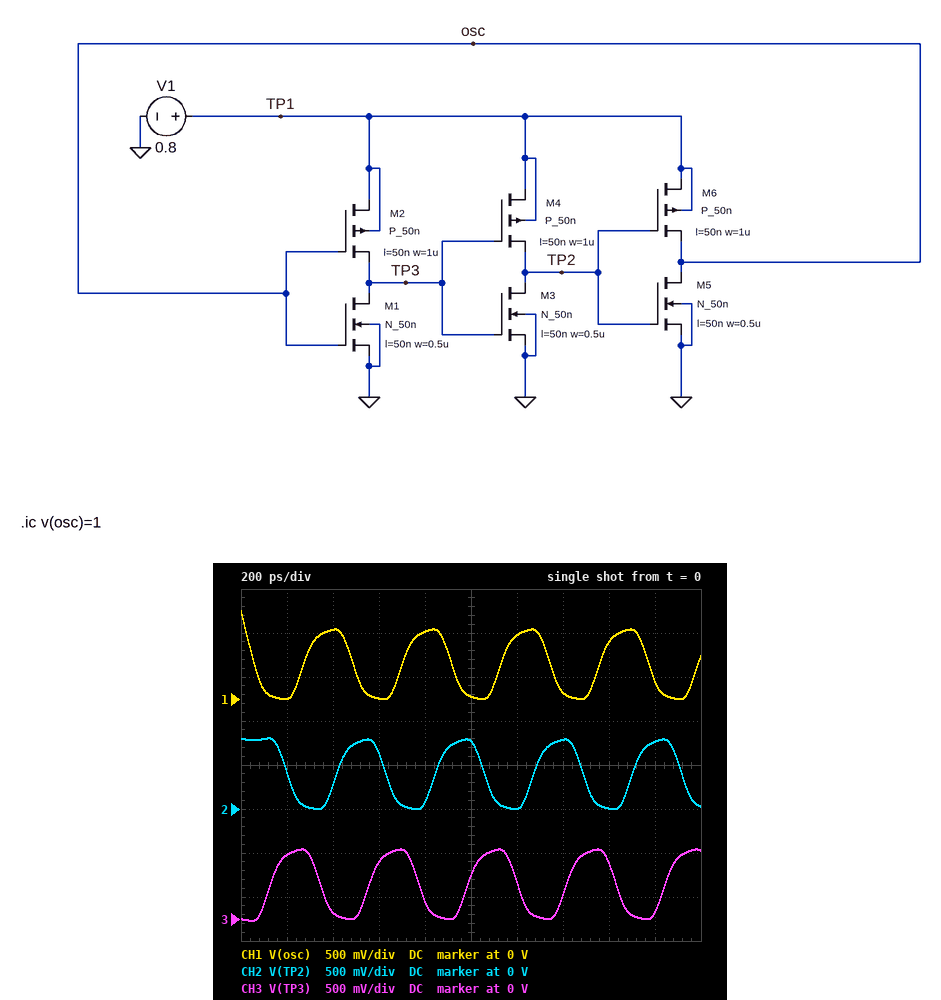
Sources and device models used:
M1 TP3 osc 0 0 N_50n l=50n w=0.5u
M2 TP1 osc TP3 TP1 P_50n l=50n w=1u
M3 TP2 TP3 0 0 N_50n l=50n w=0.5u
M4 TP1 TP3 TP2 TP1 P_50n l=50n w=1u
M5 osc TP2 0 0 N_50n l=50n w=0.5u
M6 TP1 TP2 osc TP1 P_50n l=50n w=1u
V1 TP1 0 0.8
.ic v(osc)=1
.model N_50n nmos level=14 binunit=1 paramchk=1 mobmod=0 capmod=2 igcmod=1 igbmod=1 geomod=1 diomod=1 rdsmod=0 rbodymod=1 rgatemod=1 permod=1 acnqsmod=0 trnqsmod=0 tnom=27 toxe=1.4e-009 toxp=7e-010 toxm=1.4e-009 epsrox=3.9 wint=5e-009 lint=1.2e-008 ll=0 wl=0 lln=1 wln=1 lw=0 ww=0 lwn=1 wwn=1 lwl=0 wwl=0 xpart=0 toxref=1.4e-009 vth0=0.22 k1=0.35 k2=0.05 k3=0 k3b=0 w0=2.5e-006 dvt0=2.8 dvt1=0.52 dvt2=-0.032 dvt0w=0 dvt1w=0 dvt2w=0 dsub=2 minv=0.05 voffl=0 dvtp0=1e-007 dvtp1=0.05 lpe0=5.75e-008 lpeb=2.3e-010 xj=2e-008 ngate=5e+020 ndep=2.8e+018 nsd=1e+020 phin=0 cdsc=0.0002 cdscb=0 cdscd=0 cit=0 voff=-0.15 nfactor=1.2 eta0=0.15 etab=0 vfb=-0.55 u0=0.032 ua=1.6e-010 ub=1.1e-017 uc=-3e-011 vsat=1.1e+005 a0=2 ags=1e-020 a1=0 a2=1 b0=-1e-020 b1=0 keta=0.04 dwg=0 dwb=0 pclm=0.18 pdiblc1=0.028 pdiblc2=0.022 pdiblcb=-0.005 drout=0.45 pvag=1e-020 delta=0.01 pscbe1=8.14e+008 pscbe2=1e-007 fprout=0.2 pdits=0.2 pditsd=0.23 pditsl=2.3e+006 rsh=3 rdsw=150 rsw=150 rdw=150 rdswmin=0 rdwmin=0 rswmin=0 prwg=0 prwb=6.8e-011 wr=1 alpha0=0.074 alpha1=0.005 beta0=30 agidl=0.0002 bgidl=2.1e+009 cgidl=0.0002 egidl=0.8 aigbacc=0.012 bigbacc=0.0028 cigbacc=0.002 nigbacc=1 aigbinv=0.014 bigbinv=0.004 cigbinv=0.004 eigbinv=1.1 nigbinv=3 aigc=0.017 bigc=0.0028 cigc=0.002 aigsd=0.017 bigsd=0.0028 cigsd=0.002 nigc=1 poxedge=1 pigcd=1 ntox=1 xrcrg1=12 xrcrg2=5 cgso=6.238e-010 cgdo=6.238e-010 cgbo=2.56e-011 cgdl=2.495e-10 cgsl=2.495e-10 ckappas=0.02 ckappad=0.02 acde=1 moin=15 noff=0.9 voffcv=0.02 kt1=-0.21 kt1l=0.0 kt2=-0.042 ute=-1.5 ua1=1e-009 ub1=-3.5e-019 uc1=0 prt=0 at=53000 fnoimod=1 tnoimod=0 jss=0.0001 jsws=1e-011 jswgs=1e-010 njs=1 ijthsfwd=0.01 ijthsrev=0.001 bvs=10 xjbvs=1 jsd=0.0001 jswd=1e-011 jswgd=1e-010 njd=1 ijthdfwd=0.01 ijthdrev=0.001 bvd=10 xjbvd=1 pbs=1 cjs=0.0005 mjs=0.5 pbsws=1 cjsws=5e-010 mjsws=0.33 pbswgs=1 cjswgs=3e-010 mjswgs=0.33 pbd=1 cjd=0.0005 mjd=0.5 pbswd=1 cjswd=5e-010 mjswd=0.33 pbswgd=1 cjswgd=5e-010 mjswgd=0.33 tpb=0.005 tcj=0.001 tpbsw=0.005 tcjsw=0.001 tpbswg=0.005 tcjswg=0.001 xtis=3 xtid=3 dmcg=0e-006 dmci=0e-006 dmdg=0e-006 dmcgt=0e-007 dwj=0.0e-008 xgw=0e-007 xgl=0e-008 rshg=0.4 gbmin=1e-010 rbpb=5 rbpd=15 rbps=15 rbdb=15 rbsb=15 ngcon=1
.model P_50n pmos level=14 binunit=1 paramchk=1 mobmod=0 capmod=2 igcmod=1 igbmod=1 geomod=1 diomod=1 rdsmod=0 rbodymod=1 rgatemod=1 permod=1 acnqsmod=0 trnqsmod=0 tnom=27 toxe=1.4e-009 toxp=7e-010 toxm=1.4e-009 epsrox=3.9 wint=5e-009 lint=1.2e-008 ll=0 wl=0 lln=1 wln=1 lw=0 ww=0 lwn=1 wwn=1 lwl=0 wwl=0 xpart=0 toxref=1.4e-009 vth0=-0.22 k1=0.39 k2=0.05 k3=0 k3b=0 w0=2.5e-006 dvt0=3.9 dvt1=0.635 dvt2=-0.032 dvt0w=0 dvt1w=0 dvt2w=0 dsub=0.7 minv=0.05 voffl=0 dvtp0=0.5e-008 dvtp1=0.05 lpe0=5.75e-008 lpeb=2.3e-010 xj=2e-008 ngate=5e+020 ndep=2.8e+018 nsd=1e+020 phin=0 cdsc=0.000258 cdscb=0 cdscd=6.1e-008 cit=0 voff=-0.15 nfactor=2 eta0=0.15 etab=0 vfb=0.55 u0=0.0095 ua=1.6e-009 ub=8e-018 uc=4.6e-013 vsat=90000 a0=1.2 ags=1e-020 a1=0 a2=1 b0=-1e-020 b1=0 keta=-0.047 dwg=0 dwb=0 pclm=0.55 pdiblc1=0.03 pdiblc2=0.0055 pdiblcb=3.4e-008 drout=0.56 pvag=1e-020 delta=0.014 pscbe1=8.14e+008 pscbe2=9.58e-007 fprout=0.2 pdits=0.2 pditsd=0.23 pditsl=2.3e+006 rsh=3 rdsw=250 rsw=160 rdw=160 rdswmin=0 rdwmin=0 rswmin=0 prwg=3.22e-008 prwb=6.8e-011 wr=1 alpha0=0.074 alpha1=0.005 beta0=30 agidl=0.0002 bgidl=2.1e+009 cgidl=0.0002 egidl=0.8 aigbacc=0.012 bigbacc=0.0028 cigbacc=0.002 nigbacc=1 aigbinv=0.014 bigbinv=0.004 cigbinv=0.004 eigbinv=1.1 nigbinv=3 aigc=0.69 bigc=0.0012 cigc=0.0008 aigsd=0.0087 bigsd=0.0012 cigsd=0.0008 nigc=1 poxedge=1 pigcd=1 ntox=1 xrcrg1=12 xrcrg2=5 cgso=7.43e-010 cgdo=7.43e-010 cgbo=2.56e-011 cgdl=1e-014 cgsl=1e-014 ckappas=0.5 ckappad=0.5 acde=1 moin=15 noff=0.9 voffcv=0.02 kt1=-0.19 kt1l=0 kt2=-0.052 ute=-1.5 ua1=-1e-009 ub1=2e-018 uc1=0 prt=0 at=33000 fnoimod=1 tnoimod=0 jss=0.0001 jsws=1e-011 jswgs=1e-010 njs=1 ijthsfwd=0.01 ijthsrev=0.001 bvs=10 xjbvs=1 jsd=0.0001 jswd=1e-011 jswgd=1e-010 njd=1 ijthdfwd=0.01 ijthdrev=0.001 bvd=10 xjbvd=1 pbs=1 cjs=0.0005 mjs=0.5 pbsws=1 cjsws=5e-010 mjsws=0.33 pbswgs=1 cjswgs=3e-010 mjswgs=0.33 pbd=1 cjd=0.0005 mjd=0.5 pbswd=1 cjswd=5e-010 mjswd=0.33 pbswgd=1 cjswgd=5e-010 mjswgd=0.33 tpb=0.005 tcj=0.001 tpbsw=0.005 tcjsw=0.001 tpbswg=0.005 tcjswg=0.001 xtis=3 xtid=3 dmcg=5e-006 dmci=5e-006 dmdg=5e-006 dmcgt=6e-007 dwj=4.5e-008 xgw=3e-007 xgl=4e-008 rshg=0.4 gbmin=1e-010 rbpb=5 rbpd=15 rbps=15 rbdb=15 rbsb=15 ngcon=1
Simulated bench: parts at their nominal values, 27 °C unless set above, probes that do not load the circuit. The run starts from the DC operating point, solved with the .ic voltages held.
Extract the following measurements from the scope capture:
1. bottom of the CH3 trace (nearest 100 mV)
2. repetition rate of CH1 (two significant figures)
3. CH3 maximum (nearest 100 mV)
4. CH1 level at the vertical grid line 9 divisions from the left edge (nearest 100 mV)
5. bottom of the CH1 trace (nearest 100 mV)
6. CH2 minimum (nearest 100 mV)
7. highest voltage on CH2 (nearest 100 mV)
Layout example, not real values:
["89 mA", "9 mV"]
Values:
["0 V", "2.3 GHz", "800 mV", "200 mV", "0 V", "0 V", "800 mV"]
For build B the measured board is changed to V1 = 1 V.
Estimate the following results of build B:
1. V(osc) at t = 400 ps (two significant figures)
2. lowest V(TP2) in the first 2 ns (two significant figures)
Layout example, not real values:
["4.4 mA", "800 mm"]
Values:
["82 mV", "6.3 mV"]
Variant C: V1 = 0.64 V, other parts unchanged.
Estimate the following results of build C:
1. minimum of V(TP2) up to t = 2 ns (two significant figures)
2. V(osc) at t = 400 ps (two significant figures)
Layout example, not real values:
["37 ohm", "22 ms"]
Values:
["-6.2 mV", "150 mV"]
